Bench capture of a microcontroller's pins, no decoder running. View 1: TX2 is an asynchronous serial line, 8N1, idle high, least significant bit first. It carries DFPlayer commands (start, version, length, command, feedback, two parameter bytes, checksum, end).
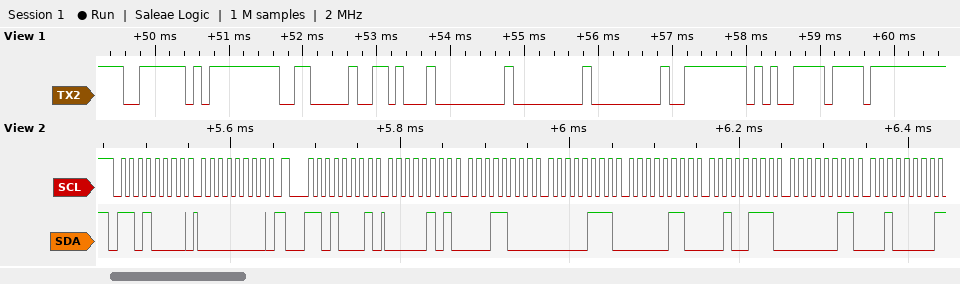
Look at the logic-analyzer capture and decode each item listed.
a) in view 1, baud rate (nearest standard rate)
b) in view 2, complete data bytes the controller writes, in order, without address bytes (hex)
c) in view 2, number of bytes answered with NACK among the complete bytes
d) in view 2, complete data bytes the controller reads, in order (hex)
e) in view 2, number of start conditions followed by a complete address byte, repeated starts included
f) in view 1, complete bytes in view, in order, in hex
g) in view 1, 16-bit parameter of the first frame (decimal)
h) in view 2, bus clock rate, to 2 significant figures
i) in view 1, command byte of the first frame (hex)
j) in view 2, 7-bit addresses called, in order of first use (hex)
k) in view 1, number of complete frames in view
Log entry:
9600 baud
00
1
05 18 07 06 27 03 20
2
0x7E 0xFF 0x06 0x16 0x00 0x00 0x00 0xFE 0xE5 0xEF
0
100 kHz
0x16
0x68
10
